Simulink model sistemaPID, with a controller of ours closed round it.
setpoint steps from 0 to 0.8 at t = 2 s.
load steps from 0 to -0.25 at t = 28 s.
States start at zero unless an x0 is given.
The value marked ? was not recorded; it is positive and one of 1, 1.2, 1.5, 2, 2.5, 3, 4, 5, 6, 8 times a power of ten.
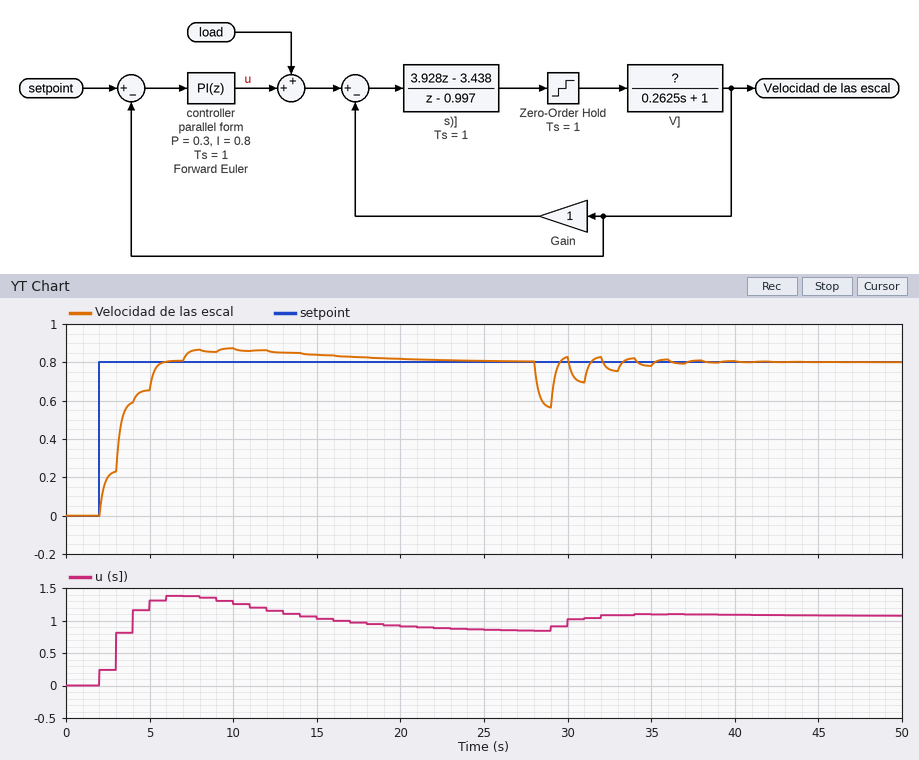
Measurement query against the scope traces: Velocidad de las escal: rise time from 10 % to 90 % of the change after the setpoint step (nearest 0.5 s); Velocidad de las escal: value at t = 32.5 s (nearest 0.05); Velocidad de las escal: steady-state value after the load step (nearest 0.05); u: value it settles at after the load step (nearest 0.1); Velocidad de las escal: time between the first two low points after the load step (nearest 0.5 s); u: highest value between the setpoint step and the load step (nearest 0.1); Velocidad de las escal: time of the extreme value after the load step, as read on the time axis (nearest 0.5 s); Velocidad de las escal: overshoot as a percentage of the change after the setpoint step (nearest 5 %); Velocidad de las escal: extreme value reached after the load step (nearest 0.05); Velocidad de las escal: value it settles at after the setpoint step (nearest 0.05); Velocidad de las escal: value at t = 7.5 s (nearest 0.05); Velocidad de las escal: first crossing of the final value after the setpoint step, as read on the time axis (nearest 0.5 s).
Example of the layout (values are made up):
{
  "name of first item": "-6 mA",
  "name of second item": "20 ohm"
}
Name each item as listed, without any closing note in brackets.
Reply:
{
  "Velocidad de las escal: rise time from 10 % to 90 % of the change after the setpoint step": "3.0 s",
  "Velocidad de las escal: value at t = 32.5 s": "0.75",
  "Velocidad de las escal: steady-state value after the load step": "0.80",
  "u: value it settles at after the load step": "1.1",
  "Velocidad de las escal: time between the first two low points after the load step": "2.0 s",
  "u: highest value between the setpoint step and the load step": "1.4",
  "Velocidad de las escal: time of the extreme value after the load step, as read on the time axis": "29.0 s",
  "Velocidad de las escal: overshoot as a percentage of the change after the setpoint step": "10 %",
  "Velocidad de las escal: extreme value reached after the load step": "0.55",
  "Velocidad de las escal: value it settles at after the setpoint step": "0.80",
  "Velocidad de las escal: value at t = 7.5 s": "0.85",
  "Velocidad de las escal: first crossing of the final value after the setpoint step, as read on the time axis": "6.0 s"
}
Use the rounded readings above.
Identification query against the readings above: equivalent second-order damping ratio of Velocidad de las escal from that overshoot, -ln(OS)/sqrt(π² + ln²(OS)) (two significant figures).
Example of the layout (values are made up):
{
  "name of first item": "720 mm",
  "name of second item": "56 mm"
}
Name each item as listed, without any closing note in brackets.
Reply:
{
  "equivalent second-order damping ratio of Velocidad de las escal from that overshoot, -ln(OS)/sqrt(π² + ln²(OS))": "0.59"
}
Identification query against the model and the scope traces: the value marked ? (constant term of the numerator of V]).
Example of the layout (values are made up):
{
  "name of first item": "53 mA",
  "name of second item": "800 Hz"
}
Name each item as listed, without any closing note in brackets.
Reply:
{
  "the value marked ?": "0.25"
}
